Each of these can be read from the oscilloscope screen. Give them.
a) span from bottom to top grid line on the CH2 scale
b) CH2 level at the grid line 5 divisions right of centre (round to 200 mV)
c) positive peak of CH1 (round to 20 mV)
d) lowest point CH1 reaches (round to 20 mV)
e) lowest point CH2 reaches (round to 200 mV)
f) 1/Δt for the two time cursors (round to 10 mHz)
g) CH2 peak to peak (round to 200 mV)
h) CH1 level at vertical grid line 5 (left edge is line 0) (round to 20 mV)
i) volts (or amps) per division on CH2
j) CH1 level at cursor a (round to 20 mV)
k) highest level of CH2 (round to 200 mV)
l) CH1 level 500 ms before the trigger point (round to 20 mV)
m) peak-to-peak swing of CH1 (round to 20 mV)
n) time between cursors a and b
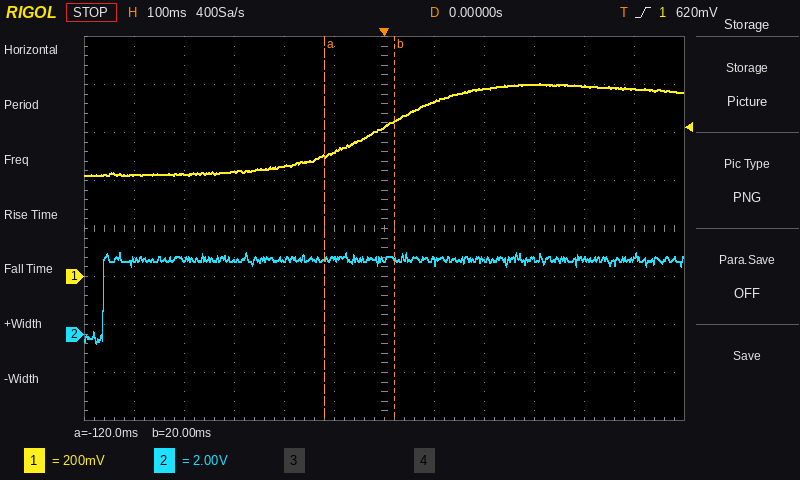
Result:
16 V
3.2 V
800 mV
420 mV
-400 mV
7.14 Hz
3.8 V
520 mV
2 V
500 mV
3.4 V
420 mV
380 mV
140 ms
